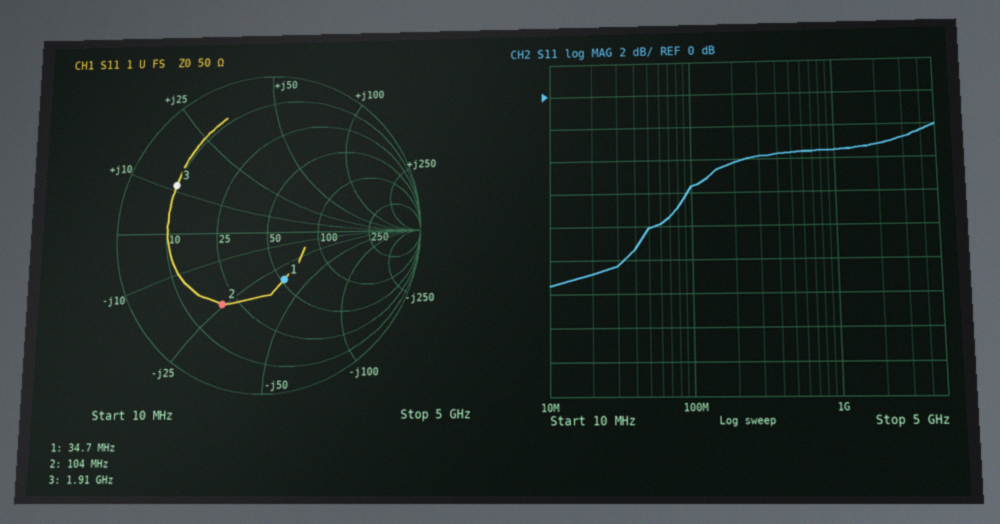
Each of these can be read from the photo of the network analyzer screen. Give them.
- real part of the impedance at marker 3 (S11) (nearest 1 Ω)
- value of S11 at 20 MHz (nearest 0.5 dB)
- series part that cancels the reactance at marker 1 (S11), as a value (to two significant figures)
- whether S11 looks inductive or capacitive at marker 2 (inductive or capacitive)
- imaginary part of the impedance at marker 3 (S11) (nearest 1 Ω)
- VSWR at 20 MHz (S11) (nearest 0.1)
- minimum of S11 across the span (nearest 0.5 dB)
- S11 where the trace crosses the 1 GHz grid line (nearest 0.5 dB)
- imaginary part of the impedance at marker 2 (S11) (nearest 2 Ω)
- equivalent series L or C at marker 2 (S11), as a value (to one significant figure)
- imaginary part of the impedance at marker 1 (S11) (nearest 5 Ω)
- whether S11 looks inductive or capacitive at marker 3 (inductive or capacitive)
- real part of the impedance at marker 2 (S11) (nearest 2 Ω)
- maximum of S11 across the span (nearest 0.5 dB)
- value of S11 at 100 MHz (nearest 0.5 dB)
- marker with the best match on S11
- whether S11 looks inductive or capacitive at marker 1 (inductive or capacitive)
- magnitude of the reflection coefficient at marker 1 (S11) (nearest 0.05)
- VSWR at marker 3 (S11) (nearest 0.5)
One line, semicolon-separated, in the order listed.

10 Ω; -11.0 dB; 160 nH; capacitive; +11 Ω; 1.8; -11.5 dB; -3.5 dB; -24 Ω; 60 pF; -35 Ω; inductive; 20 Ω; -2.0 dB; -5.5 dB; marker 1; capacitive; 0.30; 5.5
